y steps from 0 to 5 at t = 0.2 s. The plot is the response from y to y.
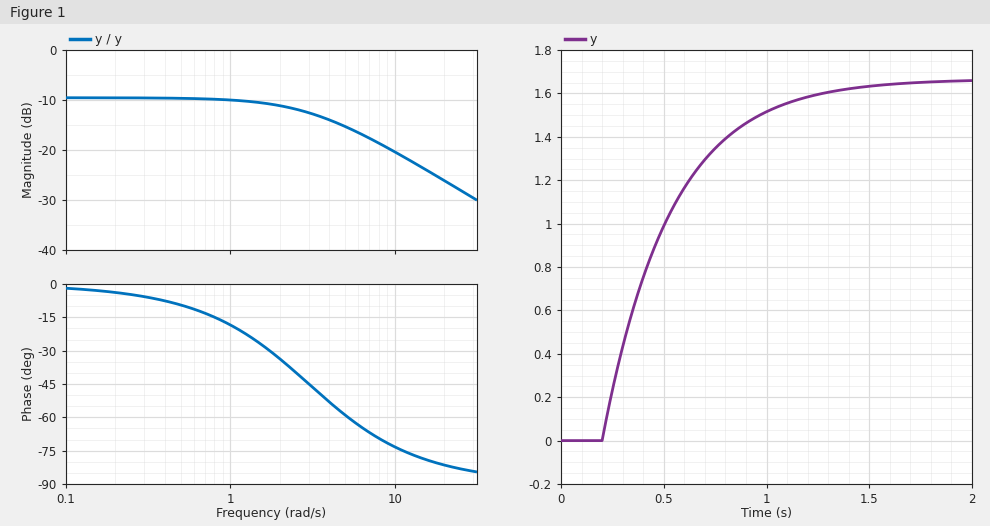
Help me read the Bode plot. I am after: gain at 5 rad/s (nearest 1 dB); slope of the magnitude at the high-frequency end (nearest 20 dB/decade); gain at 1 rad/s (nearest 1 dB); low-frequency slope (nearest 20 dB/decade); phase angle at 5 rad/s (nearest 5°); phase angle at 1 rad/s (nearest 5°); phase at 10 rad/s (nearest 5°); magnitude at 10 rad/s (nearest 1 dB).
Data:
-15 dB
-20 dB/decade
-10 dB
0 dB/decade
-60°
-20°
-75°
-20 dB
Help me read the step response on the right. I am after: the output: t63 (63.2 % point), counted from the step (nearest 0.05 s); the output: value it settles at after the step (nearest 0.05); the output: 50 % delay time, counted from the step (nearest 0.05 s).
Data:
0.35 s
1.65
0.25 s
